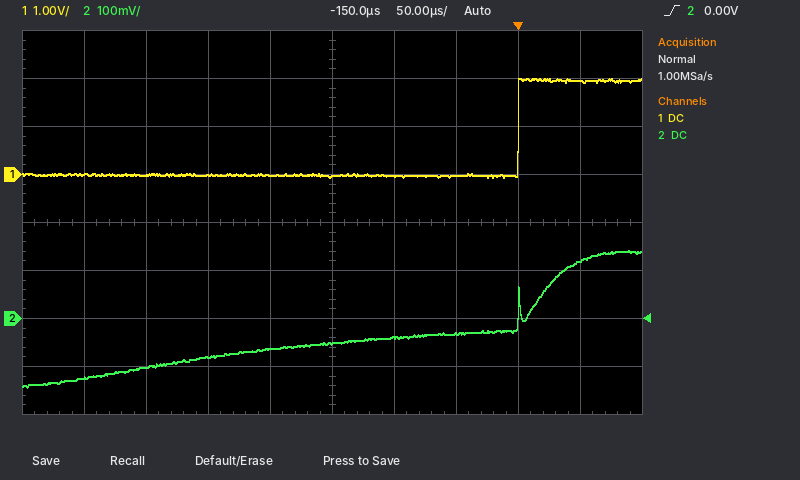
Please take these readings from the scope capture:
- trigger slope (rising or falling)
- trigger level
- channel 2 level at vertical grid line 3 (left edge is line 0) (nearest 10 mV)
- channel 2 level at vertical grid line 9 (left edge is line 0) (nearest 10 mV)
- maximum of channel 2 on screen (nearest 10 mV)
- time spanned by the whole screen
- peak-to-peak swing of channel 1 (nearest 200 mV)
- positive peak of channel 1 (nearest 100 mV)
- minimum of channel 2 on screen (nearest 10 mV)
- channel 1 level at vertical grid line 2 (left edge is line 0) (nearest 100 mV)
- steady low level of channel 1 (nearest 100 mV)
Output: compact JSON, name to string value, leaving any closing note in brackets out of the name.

{"trigger slope": "rising", "trigger level": "0.00 V", "channel 2 level at vertical grid line 3 (left edge is line 0)": "-80 mV", "channel 2 level at vertical grid line 9 (left edge is line 0)": "120 mV", "maximum of channel 2 on screen": "140 mV", "time spanned by the whole screen": "500 µs", "peak-to-peak swing of channel 1": "2.0 V", "positive peak of channel 1": "2.0 V", "minimum of channel 2 on screen": "-140 mV", "channel 1 level at vertical grid line 2 (left edge is line 0)": "0.0 V", "steady low level of channel 1": "0.0 V"}
